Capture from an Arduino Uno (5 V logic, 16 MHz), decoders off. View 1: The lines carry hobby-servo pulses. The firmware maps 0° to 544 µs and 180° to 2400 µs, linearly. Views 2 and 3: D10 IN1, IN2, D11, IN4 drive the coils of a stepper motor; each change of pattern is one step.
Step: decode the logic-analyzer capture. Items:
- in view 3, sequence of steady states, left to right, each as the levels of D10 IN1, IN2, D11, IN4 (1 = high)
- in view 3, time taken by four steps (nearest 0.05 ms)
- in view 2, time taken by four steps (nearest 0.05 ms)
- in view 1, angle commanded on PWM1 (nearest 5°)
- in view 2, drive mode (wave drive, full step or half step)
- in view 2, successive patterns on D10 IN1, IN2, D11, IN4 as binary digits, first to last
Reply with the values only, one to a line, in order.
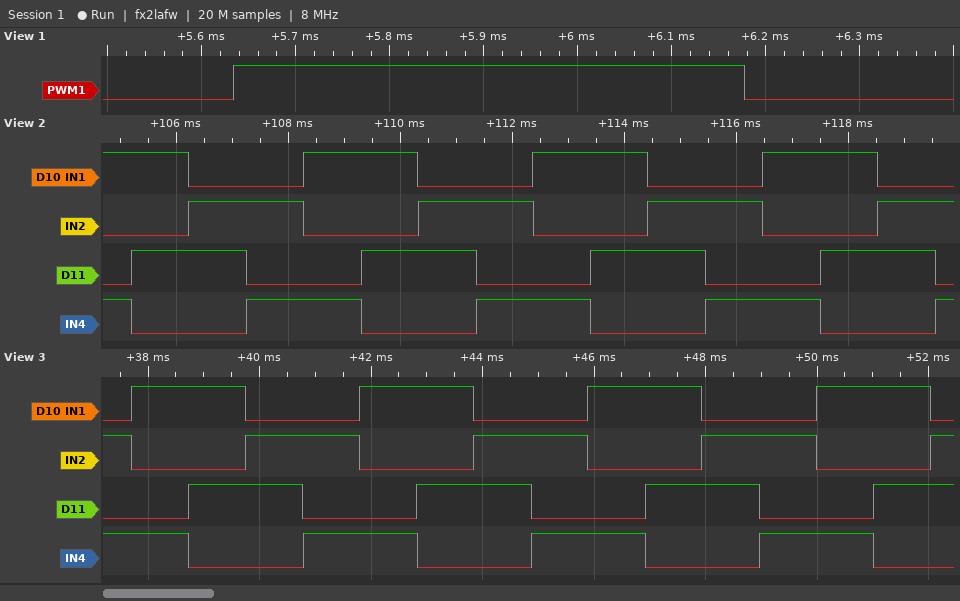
0101 1001 1010 0110 0101 1001 1010 0110 0101 1001 1010 0110 0101 1001 1010 0110
4.10 ms
4.10 ms
0°
full step
1001 1010 0110 0101 1001 1010 0110 0101 1001 1010 0110 0101 1001 1010 0110 0101
